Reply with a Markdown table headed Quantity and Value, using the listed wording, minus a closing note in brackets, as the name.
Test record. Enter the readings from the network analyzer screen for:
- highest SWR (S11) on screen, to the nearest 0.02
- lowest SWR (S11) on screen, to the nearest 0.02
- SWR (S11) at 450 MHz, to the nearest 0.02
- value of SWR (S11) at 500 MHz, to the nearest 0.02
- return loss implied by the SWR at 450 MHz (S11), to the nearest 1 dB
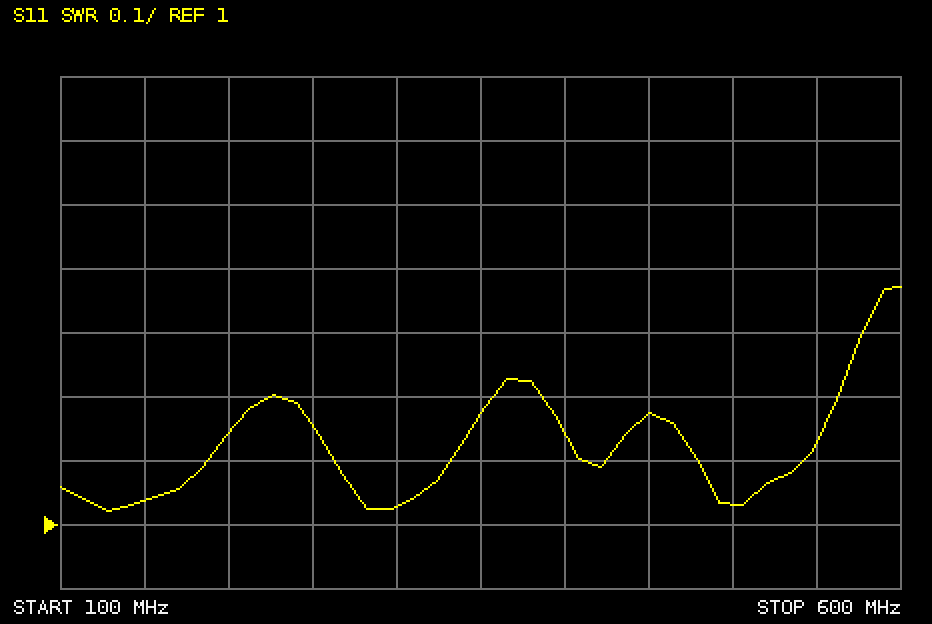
| Quantity | Value |
|---|---|
| highest SWR (S11) on screen, to the nearest 0.02 | 1.38 |
| lowest SWR (S11) on screen, to the nearest 0.02 | 1.02 |
| SWR (S11) at 450 MHz, to the nearest 0.02 | 1.18 |
| value of SWR (S11) at 500 MHz, to the nearest 0.02 | 1.04 |
| return loss implied by the SWR at 450 MHz (S11), to the nearest 1 dB | 22 dB |
